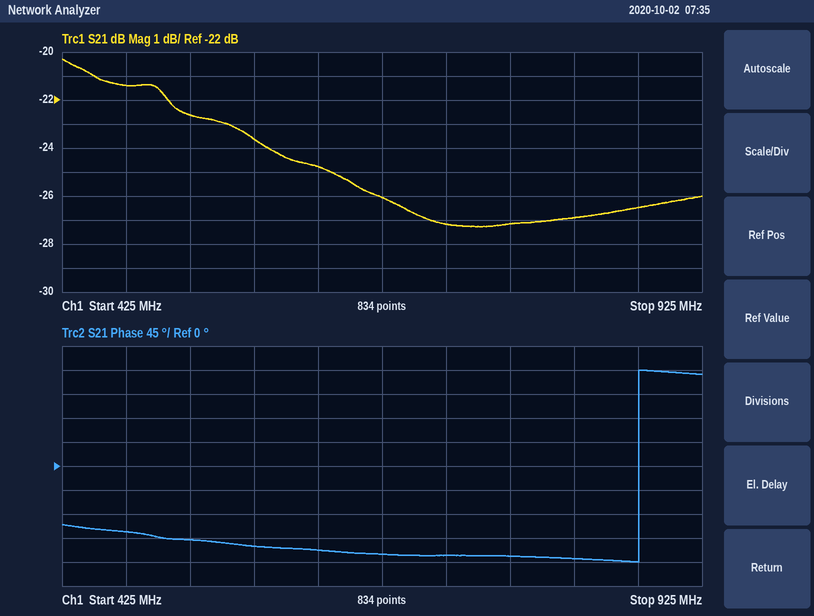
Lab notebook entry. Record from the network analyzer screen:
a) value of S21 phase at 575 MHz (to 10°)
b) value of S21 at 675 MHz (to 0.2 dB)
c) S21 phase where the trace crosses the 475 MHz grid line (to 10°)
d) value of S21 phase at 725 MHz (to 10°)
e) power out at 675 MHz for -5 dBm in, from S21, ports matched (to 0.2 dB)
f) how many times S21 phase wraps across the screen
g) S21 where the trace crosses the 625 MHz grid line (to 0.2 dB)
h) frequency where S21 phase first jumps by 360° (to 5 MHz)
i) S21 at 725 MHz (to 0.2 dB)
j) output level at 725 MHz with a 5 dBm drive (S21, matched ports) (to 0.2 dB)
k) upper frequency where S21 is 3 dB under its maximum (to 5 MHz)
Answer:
-150°
-26.0 dB
-120°
-170°
-31.0 dBm
1
-24.8 dB
875 MHz
-27.2 dB
-22.2 dBm
565 MHz
